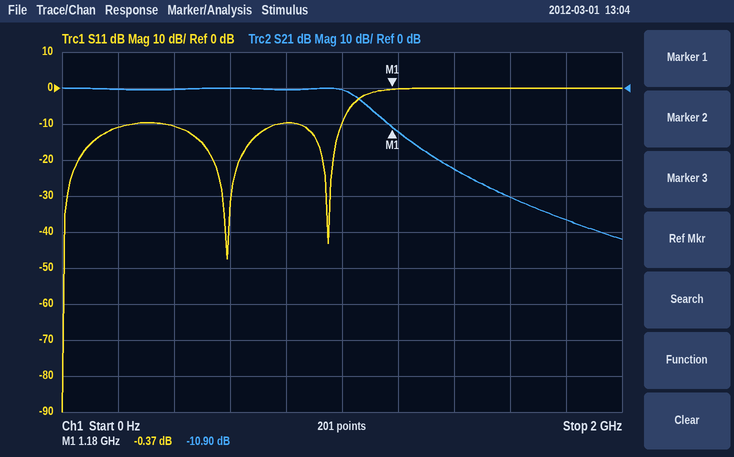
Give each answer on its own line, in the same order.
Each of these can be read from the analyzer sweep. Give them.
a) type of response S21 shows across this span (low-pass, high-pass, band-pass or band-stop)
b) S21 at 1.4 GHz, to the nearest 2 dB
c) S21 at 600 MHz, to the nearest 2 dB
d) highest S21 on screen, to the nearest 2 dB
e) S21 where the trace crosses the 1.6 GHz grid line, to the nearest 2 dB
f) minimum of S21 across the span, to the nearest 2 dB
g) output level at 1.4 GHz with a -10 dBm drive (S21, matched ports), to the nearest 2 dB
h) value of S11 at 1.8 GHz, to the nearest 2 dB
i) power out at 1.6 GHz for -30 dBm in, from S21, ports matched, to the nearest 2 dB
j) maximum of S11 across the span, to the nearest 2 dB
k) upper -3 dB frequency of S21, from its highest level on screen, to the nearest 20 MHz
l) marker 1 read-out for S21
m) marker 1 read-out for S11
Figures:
low-pass
-22 dB
0 dB
0 dB
-30 dB
-42 dB
-32 dBm
0 dB
-60 dBm
0 dB
1.06 GHz
-10.90 dB
-0.37 dB
